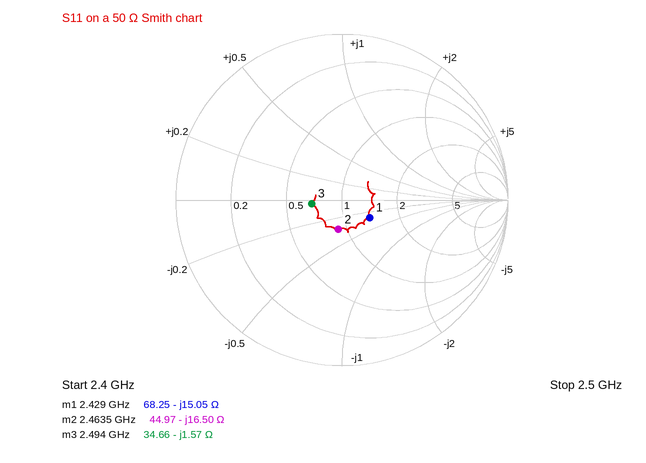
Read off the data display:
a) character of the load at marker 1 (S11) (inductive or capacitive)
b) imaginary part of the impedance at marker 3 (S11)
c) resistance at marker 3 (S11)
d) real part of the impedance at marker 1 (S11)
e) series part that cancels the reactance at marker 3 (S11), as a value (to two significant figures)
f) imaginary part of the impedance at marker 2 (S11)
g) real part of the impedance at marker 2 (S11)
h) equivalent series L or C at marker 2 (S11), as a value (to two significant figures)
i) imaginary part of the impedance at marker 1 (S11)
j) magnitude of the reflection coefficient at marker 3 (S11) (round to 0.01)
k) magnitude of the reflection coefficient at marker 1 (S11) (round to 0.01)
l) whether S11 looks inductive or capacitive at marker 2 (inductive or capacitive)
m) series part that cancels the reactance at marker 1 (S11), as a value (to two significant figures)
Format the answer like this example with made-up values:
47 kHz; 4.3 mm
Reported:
capacitive; -1.57 Ω; 34.66 Ω; 68.25 Ω; 100 pH; -16.50 Ω; 44.97 Ω; 3.9 pF; -15.05 Ω; 0.18; 0.20; capacitive; 990 pH
